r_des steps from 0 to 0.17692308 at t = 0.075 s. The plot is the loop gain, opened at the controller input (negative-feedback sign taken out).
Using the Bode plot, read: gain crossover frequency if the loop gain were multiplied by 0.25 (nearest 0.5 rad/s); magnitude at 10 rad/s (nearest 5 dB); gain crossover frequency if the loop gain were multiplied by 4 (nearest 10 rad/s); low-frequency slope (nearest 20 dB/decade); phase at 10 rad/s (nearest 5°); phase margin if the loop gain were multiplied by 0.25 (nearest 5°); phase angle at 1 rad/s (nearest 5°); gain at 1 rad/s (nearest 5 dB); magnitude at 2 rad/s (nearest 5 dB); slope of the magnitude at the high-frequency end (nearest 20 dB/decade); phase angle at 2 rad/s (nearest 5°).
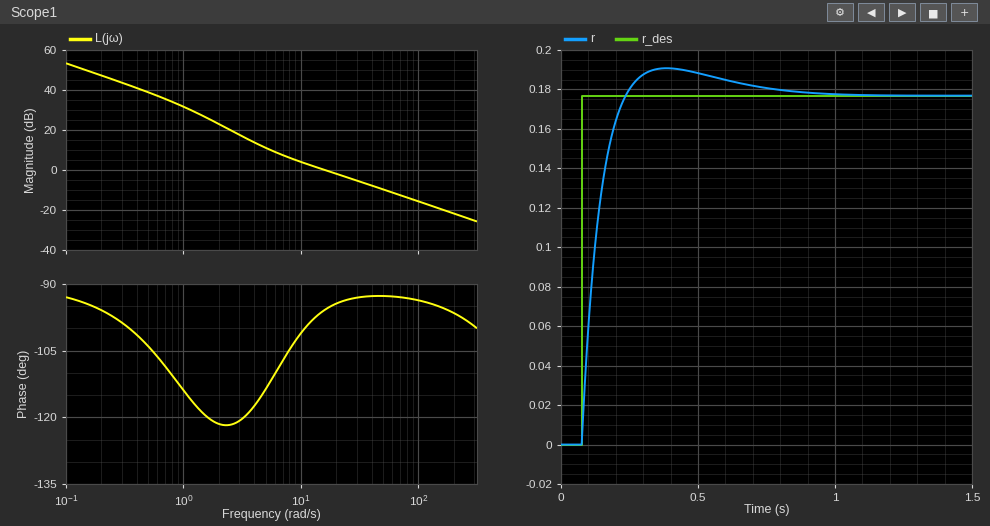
4.5 rad/s
5 dB
70 rad/s
-20 dB/decade
-100°
65°
-115°
30 dB
25 dB
-20 dB/decade
-120°
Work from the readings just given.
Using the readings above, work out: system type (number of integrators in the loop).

1
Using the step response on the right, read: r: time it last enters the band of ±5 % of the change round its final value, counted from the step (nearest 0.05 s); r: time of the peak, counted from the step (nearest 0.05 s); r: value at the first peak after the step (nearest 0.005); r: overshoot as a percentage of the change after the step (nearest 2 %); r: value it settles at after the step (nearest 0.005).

0.50 s
0.30 s
0.190
8 %
0.175
